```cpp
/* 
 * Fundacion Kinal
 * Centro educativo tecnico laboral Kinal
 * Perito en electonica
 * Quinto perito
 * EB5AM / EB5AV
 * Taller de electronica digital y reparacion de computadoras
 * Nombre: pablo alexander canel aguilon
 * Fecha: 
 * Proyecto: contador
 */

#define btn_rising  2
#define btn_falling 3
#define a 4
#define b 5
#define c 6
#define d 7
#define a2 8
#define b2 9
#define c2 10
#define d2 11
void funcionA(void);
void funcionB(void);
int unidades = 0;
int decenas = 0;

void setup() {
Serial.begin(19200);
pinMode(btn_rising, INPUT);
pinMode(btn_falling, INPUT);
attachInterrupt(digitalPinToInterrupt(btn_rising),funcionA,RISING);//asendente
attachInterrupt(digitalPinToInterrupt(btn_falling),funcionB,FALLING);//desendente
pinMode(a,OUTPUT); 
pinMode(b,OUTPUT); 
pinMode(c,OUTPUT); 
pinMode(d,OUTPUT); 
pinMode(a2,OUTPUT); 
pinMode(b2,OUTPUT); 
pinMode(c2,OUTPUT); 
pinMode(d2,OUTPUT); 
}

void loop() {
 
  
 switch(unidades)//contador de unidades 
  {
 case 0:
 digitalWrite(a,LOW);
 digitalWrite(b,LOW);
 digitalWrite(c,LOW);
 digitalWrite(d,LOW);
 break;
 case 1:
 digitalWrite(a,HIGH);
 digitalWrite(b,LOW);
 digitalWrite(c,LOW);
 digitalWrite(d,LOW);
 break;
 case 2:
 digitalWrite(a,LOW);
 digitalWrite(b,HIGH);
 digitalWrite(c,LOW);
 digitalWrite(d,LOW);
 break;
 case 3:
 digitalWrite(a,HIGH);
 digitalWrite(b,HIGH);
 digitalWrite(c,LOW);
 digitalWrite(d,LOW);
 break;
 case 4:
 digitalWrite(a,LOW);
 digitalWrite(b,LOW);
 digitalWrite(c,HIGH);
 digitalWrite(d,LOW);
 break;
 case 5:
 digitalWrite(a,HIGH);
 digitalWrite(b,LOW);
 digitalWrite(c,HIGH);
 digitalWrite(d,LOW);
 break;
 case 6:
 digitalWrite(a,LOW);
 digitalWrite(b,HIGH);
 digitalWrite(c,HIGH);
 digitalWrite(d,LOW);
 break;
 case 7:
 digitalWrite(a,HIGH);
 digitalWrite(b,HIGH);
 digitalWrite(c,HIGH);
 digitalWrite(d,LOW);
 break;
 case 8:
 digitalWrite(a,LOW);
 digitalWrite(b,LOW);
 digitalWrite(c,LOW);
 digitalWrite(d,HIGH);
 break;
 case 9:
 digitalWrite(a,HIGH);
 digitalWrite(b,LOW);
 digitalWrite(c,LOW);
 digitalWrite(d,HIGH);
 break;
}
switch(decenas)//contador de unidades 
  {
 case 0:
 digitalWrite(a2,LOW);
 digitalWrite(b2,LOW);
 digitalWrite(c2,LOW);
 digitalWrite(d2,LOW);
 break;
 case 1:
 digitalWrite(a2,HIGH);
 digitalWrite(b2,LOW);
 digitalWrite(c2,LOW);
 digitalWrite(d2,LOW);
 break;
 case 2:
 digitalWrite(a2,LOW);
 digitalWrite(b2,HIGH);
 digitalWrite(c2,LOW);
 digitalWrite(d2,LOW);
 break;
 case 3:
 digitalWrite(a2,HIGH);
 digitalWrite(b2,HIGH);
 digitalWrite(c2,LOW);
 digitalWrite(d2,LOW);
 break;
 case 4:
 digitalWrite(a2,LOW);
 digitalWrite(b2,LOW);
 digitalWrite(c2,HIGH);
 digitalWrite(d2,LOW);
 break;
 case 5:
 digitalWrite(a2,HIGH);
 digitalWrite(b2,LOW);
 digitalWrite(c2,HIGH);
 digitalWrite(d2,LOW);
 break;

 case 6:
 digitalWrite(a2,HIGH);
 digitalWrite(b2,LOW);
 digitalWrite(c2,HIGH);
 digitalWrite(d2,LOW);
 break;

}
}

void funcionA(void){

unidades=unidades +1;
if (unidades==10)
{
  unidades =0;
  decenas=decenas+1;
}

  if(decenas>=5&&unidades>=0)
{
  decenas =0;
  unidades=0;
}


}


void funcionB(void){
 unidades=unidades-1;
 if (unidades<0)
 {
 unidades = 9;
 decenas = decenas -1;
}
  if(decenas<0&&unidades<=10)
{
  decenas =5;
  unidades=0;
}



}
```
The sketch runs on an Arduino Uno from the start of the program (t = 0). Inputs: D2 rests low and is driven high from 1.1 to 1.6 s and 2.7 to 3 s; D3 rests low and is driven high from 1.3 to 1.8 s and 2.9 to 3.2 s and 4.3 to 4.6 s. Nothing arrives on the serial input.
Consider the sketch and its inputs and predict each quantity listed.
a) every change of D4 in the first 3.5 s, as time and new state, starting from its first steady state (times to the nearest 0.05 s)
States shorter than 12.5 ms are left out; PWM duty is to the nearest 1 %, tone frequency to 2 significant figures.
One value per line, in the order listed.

0 s low; 1.1 s high; 1.8 s low; 2.7 s high; 3.2 s low
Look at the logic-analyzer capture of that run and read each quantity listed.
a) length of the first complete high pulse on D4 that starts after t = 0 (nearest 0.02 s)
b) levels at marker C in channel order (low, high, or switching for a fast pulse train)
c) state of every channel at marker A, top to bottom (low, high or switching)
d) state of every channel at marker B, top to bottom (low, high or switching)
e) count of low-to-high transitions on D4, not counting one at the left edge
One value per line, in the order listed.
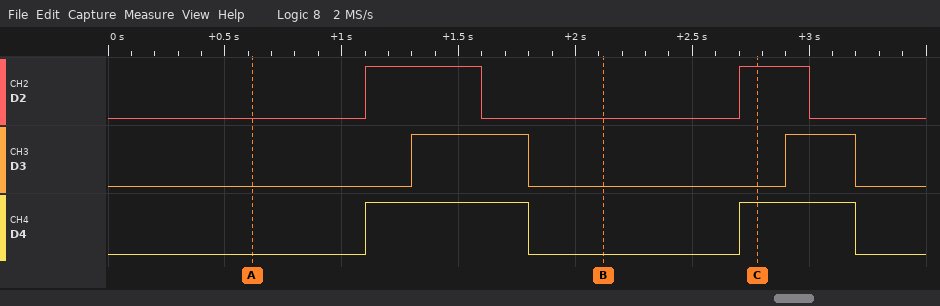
0.70 s
D2 high, D3 low, D4 high
D2 low, D3 low, D4 low
D2 low, D3 low, D4 low
2
